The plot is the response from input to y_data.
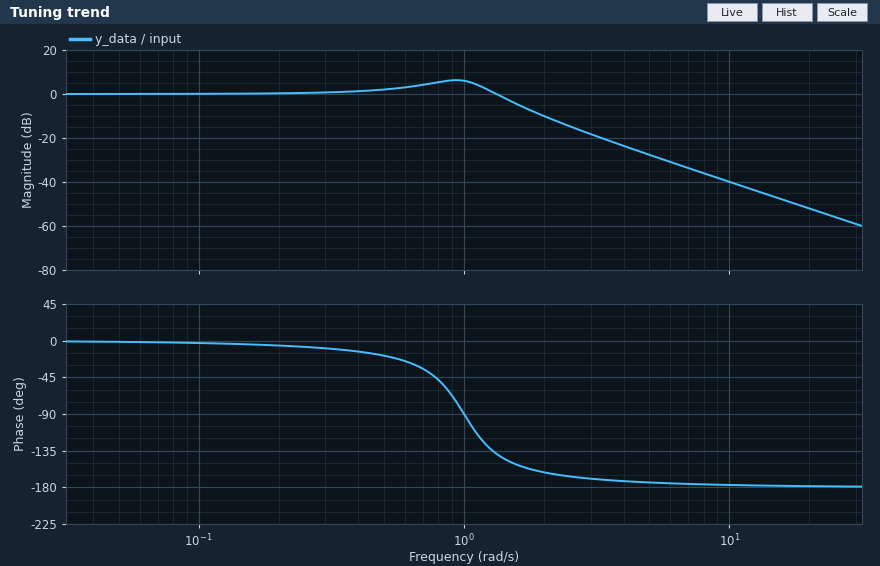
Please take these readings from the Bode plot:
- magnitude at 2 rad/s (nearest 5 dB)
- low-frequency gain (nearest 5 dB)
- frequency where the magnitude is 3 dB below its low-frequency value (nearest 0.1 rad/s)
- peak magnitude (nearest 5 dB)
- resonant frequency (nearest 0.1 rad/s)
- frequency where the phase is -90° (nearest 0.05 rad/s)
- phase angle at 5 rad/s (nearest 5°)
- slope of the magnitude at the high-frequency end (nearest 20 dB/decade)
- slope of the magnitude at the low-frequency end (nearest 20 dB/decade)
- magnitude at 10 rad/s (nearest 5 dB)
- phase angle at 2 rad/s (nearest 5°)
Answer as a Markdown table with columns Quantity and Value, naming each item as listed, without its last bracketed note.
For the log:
| Quantity | Value |
|---|---|
| magnitude at 2 rad/s | -10 dB |
| low-frequency gain | 0 dB |
| frequency where the magnitude is 3 dB below its low-frequency value | 1.5 rad/s |
| peak magnitude | 5 dB |
| resonant frequency | 0.9 rad/s |
| frequency where the phase is -90° | 1.00 rad/s |
| phase angle at 5 rad/s | -175° |
| slope of the magnitude at the high-frequency end | -40 dB/decade |
| slope of the magnitude at the low-frequency end | 0 dB/decade |
| magnitude at 10 rad/s | -40 dB |
| phase angle at 2 rad/s | -160° |
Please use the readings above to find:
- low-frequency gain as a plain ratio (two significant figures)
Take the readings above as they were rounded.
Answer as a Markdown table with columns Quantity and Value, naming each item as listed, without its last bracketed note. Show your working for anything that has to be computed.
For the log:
| Quantity | Value |
|---|---|
| low-frequency gain as a plain ratio | 10^(0 / 20) = 1.0 |
